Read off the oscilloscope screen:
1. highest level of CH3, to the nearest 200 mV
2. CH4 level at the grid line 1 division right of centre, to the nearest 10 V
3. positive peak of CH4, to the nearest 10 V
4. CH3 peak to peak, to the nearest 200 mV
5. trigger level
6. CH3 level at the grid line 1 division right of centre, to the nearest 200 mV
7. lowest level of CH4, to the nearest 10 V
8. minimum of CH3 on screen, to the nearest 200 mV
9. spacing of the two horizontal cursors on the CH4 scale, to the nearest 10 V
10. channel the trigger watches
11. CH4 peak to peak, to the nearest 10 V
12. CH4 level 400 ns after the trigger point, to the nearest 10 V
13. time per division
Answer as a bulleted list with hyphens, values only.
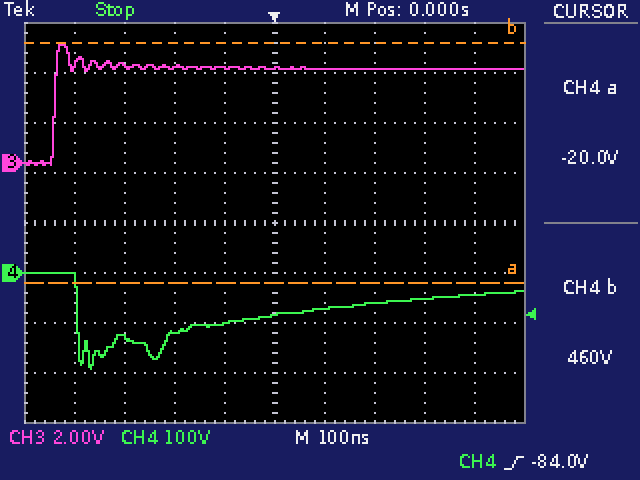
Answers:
- 4.8 V
- -70 V
- 0 V
- 4.8 V
- -84.0 V
- 3.8 V
- -190 V
- 0.0 V
- 480 V
- CH4
- 190 V
- -40 V
- 100 ns
